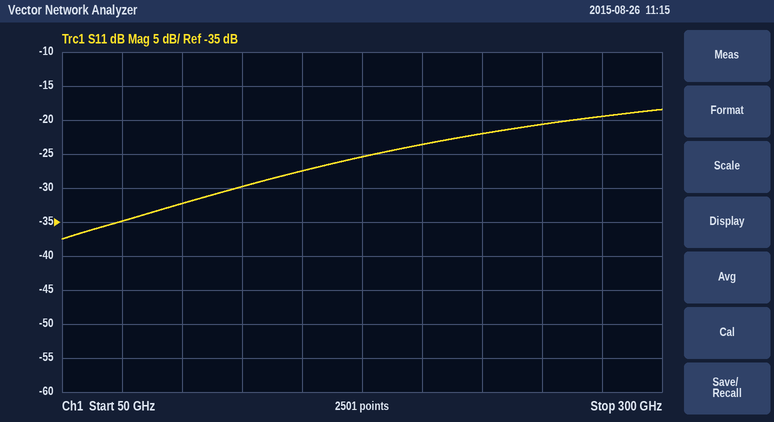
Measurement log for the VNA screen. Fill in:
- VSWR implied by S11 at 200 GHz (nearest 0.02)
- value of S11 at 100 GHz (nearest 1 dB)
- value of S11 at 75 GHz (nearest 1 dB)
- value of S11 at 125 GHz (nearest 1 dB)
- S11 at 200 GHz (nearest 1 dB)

1.14
-32 dB
-35 dB
-30 dB
-24 dB
